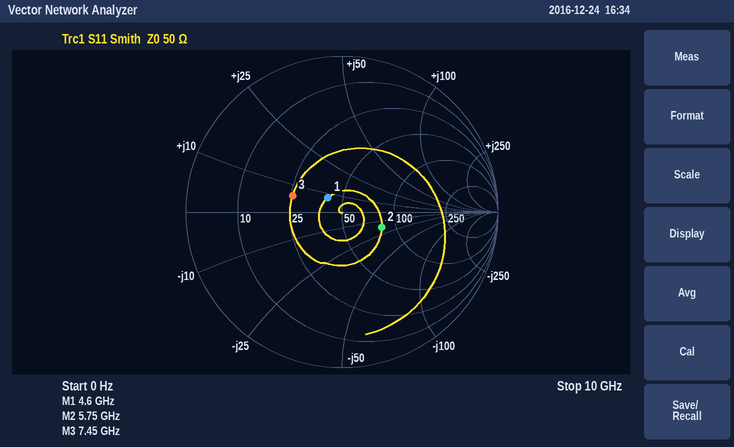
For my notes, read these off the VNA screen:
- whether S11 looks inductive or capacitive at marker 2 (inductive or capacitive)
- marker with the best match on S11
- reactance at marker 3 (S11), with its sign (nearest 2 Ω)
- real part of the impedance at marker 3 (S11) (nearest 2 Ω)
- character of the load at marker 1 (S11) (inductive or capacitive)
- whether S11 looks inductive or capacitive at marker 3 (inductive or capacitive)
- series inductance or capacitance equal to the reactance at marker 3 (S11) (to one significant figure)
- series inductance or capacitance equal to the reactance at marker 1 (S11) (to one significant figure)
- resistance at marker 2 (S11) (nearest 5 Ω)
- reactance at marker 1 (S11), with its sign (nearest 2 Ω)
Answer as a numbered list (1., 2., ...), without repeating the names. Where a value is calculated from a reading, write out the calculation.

1. capacitive
2. marker 1
3. +6 Ω
4. 26 Ω
5. inductive
6. inductive
7. L = 6 Ω/(2π × 7.45 GHz) ≈ 128 pH, so 100 pH to one significant figure
8. L = 8 Ω/(2π × 4.6 GHz) ≈ 277 pH, so 300 pH to one significant figure
9. 80 Ω
10. +8 Ω
